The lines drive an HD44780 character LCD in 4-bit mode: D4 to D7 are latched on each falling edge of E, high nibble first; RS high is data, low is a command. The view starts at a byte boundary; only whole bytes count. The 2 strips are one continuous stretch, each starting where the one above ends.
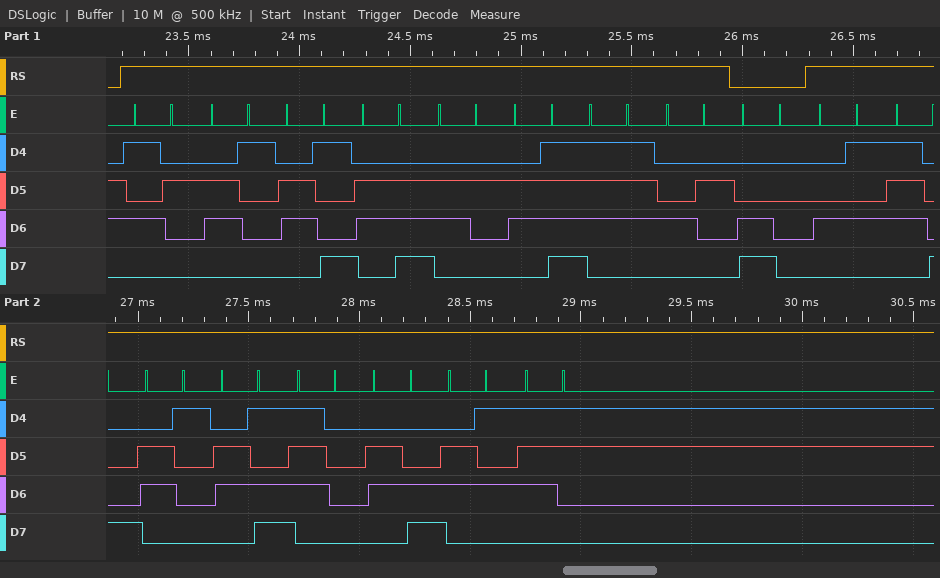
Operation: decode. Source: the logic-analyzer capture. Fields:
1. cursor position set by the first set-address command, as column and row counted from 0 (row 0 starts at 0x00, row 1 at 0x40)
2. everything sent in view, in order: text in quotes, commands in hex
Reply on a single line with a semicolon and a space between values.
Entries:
column 0, row 1; "RainbowB" 0xC0 "Examples"
